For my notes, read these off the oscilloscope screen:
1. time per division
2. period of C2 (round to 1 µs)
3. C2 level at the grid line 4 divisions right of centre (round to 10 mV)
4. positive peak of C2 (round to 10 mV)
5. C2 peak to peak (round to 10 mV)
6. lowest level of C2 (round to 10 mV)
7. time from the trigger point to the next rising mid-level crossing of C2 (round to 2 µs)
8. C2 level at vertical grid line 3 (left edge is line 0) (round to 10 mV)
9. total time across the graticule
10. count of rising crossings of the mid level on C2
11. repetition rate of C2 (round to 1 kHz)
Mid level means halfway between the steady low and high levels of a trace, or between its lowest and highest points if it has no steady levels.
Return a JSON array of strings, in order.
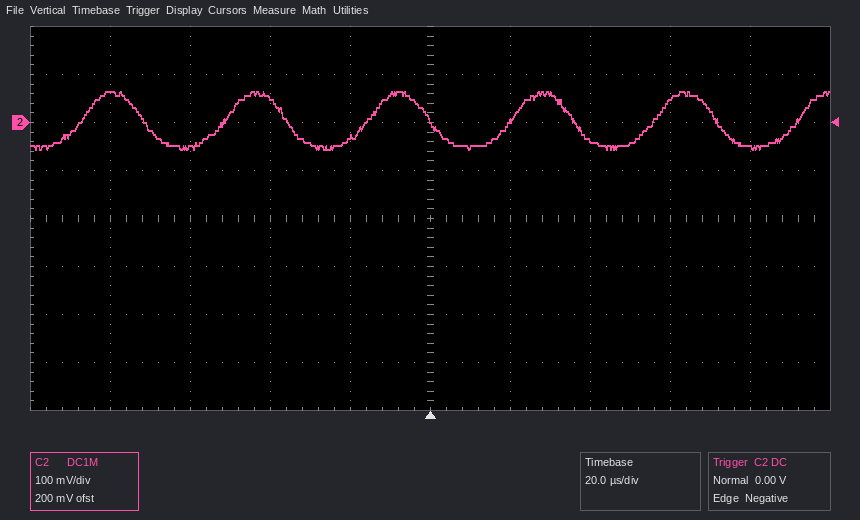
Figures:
["20 µs", "36 µs", "-50 mV", "60 mV", "120 mV", "-60 mV", "20 µs", "50 mV", "200 µs", "6", "28 kHz"]
